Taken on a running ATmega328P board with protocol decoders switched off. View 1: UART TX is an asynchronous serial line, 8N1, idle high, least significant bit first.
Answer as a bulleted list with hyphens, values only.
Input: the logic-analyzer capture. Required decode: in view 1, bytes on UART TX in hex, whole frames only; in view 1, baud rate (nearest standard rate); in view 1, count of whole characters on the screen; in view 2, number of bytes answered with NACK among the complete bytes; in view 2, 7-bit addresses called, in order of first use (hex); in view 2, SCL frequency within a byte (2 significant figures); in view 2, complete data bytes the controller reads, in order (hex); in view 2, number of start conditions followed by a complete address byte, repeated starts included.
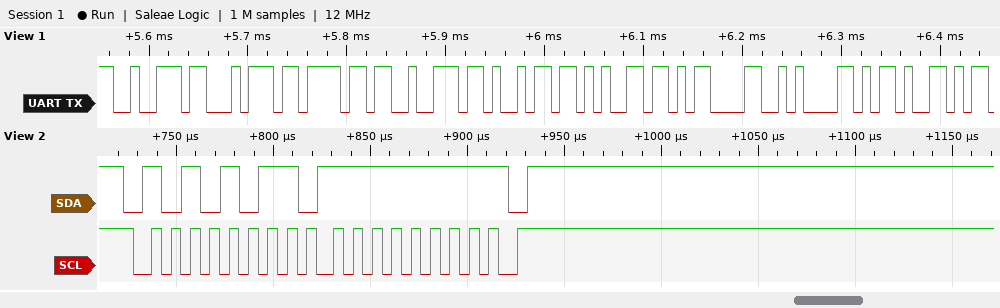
- 72 74 6F 72 69 65 0D 0A 2D
- 115200 baud
- 9
- 1
- 0x55
- 100 kHz
- FF
- 1
